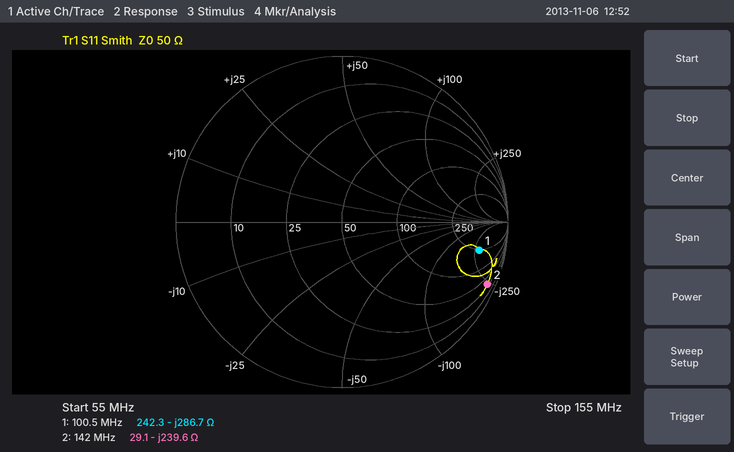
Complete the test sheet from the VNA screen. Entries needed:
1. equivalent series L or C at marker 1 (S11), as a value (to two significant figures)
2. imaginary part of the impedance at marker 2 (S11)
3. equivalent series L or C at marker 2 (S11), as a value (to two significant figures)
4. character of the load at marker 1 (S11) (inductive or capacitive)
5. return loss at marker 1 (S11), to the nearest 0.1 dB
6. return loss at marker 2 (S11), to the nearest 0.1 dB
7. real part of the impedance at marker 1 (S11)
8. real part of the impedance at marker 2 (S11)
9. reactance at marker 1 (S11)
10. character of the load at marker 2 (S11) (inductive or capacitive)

5.5 pF
-239.6 Ω
4.7 pF
capacitive
1.5 dB
0.4 dB
242.3 Ω
29.1 Ω
-286.7 Ω
capacitive
